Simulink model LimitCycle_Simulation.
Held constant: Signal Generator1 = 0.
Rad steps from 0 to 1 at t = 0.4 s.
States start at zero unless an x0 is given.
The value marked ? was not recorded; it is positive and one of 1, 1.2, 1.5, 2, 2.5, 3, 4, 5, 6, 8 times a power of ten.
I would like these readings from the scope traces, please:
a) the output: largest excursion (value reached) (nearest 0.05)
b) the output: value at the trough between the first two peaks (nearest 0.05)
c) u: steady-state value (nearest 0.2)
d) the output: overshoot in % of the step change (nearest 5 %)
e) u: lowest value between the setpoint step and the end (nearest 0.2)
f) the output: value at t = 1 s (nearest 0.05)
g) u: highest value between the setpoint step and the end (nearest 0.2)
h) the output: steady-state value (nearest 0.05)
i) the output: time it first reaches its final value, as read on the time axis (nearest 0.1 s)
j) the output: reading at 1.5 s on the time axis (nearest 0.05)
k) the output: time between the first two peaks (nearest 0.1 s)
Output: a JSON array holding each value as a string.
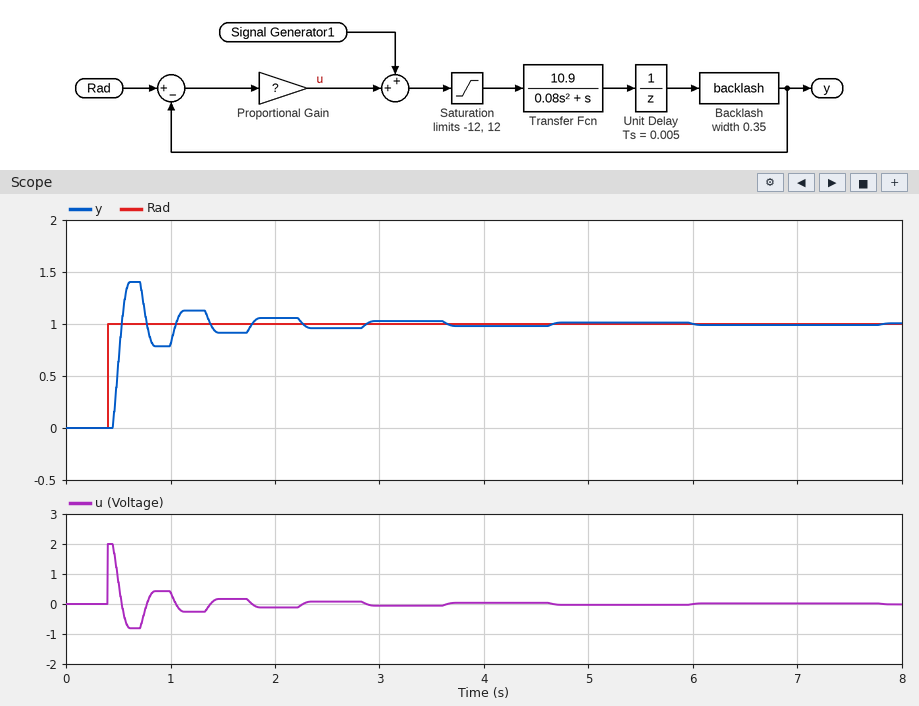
["1.40", "0.80", "0.0", "40 %", "-0.8", "0.80", "2.0", "1.00", "0.5 s", "0.90", "0.6 s"]
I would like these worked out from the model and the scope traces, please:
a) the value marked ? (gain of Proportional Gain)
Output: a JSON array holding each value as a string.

["2"]
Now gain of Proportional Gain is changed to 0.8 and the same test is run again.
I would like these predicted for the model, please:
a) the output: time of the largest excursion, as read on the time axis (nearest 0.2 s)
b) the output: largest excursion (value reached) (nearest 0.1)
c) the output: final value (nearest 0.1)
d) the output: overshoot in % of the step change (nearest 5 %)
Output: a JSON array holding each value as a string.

["0.8 s", "1.1", "1.0", "15 %"]
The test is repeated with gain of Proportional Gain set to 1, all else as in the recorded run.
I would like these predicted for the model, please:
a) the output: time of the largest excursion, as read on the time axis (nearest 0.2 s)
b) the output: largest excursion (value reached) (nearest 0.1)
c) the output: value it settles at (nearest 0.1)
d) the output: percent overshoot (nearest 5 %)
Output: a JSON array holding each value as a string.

["0.8 s", "1.2", "1.0", "20 %"]
